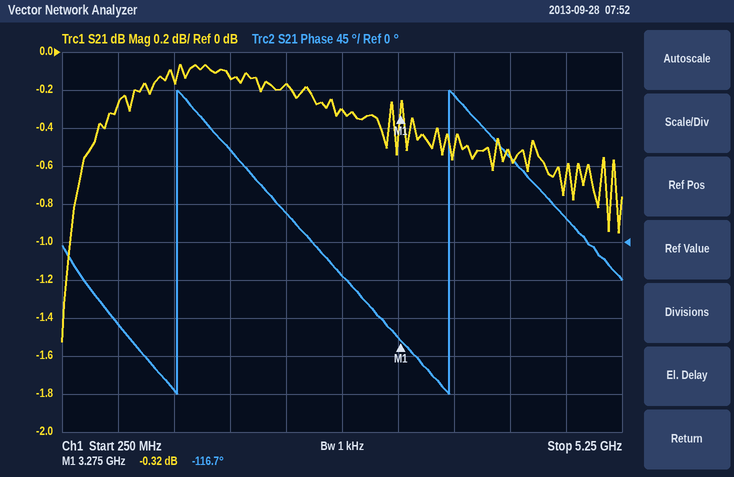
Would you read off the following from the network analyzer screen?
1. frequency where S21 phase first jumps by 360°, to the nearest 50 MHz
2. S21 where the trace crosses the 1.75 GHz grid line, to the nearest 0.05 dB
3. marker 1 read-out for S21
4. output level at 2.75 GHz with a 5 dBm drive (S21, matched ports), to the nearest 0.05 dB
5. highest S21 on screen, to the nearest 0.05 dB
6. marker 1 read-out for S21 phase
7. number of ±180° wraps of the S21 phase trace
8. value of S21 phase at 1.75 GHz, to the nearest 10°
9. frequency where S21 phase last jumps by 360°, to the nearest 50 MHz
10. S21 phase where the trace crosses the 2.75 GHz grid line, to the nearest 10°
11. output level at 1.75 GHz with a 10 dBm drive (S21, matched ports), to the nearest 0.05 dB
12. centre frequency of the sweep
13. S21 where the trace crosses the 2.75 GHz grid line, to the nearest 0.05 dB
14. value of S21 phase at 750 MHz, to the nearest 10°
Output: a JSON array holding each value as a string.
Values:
["1.30 GHz", "-0.15 dB", "-0.32 dB", "4.70 dBm", "-0.05 dB", "-116.7°", "2", "110°", "3.70 GHz", "-40°", "9.85 dBm", "2.75 GHz", "-0.30 dB", "-100°"]
